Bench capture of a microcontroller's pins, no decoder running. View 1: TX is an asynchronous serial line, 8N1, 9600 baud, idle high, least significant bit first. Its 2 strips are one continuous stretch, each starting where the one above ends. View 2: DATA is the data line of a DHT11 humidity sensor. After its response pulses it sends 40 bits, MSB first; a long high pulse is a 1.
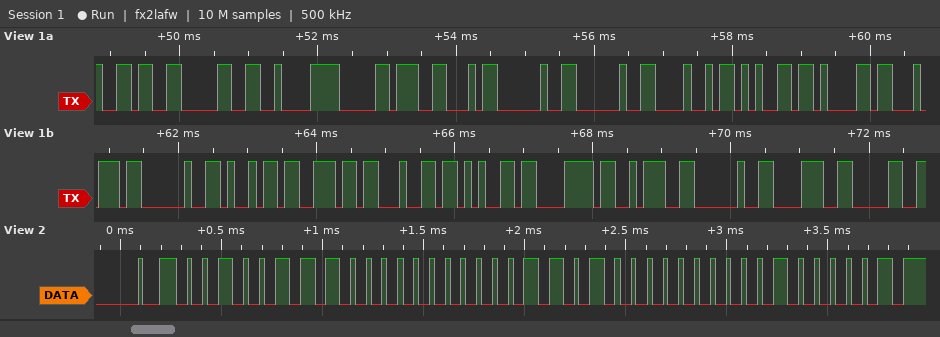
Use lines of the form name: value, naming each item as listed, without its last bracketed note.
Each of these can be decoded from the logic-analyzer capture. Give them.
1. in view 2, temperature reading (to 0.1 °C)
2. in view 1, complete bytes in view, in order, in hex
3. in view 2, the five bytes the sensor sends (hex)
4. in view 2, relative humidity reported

in view 2, temperature reading: 26.0 °C
in view 1, complete bytes in view, in order, in hex: 0x36 0x30 0xC2 0xB0 0x46 0x20 0x20 0x48 0x65 0x61 0x74 0x20 0x69 0x6E 0x64 0x65 0x78 0x3A 0x20 0x38 0x30
in view 2, the five bytes the sensor sends: 27 00 1A 00 41
in view 2, relative humidity reported: 39 %
